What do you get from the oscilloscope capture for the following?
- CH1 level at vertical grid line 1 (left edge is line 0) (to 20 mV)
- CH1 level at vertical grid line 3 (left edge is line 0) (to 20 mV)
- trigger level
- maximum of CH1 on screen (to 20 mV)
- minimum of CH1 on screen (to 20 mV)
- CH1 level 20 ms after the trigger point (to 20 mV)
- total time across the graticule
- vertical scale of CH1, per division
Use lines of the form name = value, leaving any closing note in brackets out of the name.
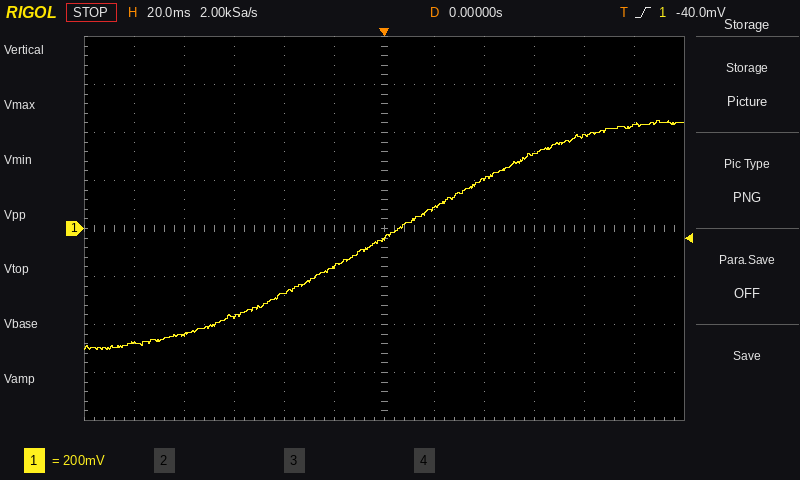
CH1 level at vertical grid line 1 (left edge is line 0) = -480 mV
CH1 level at vertical grid line 3 (left edge is line 0) = -360 mV
trigger level = -40.0 mV
maximum of CH1 on screen = 440 mV
minimum of CH1 on screen = -500 mV
CH1 level 20 ms after the trigger point = 80 mV
total time across the graticule = 240 ms
vertical scale of CH1, per division = 200 mV
